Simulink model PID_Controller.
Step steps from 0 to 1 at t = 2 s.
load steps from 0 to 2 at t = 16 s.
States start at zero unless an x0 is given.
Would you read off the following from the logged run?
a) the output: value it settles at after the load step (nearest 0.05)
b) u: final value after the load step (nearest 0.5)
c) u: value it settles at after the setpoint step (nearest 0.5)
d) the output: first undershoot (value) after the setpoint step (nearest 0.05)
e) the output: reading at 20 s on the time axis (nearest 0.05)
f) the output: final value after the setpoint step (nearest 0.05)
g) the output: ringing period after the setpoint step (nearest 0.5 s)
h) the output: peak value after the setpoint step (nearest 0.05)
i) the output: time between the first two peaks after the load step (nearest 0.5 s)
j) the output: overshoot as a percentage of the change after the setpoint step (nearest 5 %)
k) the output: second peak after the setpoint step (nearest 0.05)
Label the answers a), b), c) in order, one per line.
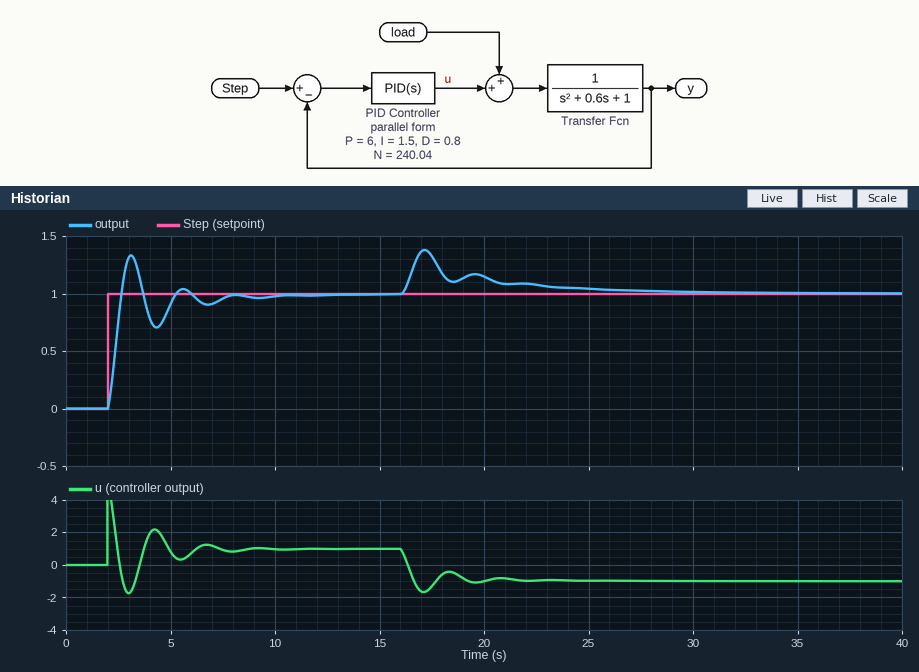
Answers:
a) 1.00
b) -1.0
c) 1.0
d) 0.70
e) 1.15
f) 1.00
g) 2.5 s
h) 1.35
i) 2.5 s
j) 35 %
k) 1.05
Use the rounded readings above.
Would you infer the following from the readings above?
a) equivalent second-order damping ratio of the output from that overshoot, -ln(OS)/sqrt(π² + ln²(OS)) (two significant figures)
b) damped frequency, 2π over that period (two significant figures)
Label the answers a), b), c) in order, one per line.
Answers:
a) 0.32
b) 2.5 rad/s
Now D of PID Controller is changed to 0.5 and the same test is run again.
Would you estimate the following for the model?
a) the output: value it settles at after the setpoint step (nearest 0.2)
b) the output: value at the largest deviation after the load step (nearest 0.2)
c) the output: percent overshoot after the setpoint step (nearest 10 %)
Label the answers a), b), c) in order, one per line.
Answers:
a) 1.0
b) 1.4
c) 40 %
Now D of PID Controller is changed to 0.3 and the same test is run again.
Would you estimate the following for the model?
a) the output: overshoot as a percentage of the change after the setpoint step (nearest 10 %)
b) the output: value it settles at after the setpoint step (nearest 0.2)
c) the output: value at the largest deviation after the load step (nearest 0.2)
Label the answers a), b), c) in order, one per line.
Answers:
a) 50 %
b) 1.0
c) 1.4
